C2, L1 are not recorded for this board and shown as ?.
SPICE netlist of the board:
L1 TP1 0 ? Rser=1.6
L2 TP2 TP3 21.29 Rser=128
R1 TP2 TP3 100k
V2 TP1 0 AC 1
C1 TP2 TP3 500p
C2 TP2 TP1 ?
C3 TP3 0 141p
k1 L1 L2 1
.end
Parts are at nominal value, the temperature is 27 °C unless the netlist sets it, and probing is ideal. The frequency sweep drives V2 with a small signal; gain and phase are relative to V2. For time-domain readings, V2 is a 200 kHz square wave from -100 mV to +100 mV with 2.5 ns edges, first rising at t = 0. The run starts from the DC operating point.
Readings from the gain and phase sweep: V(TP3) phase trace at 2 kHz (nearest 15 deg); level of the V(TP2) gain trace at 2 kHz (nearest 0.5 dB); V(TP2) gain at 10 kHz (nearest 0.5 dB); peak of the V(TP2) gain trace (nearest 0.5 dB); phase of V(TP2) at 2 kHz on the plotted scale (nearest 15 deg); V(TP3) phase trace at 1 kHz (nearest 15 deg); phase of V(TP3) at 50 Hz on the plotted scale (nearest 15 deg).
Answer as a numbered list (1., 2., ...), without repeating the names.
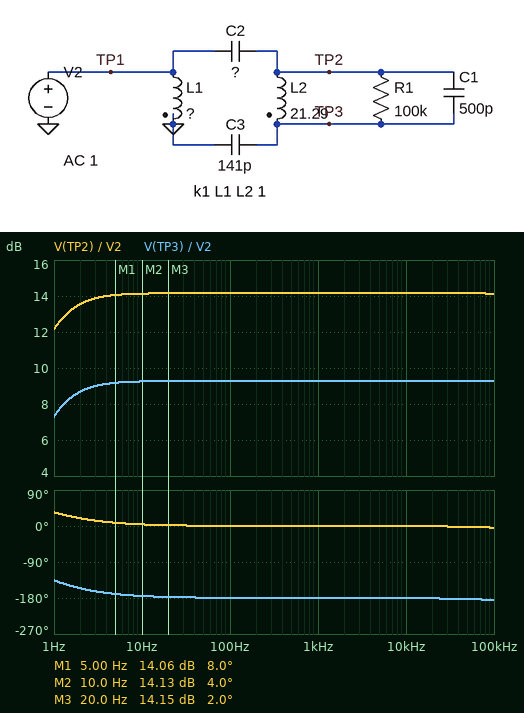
1. -180 deg
2. 14.0 dB
3. 14.0 dB
4. 14.0 dB
5. 0 deg
6. -180 deg
7. -180 deg
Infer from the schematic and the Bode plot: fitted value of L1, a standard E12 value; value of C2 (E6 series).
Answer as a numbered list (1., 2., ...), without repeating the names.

1. 330 mH
2. 100 pF
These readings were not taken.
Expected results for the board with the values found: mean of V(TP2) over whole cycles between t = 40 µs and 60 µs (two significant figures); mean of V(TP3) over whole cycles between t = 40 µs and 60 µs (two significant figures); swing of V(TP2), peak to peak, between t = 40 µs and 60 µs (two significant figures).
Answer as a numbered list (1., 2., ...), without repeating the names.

1. 510 mV
2. -290 mV
3. 1.0 V
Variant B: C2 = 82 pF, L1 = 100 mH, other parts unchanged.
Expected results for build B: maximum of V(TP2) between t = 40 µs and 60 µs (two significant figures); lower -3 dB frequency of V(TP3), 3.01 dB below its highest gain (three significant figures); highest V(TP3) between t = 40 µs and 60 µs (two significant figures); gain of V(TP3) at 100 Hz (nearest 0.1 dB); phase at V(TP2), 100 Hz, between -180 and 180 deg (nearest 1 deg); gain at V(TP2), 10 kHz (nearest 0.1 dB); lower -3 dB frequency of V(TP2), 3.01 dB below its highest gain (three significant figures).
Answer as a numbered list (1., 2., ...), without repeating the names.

1. 1.9 V
2. 2.52 Hz
3. 62 mV
4. 13.9 dB
5. 1 deg
6. 19.6 dB
7. 2.53 Hz
